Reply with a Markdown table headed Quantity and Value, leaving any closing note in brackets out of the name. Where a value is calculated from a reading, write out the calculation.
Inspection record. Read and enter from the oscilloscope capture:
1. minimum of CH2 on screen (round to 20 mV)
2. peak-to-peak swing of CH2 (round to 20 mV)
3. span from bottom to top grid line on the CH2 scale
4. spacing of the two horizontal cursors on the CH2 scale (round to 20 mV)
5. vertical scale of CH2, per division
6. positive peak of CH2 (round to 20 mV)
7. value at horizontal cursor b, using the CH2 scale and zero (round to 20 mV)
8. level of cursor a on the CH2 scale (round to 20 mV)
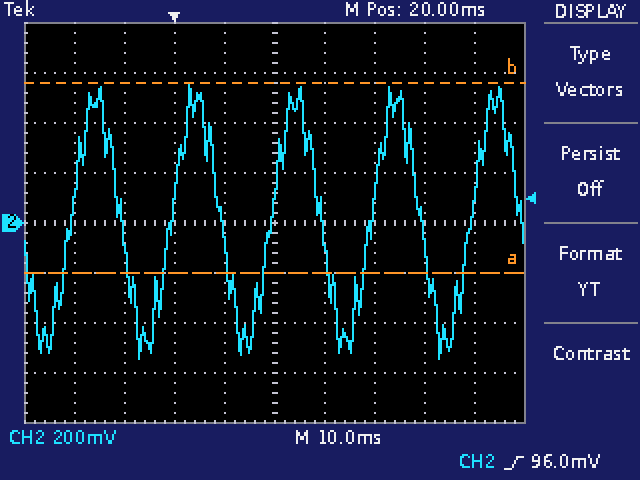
| Quantity | Value |
|---|---|
| minimum of CH2 on screen | -540 mV |
| peak-to-peak swing of CH2 | 560 mV − (-540 mV) = 1.10 V |
| span from bottom to top grid line on the CH2 scale | 1.6 V |
| spacing of the two horizontal cursors on the CH2 scale | 760 mV |
| vertical scale of CH2, per division | 200 mV |
| positive peak of CH2 | 560 mV |
| value at horizontal cursor b, using the CH2 scale and zero | 560 mV |
| level of cursor a on the CH2 scale | -200 mV |
